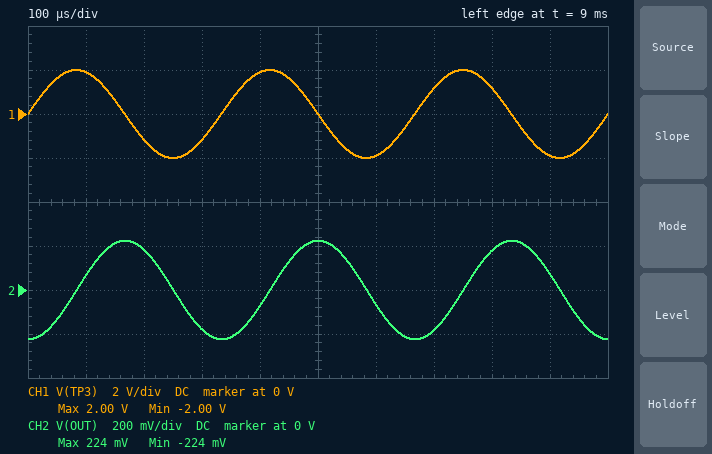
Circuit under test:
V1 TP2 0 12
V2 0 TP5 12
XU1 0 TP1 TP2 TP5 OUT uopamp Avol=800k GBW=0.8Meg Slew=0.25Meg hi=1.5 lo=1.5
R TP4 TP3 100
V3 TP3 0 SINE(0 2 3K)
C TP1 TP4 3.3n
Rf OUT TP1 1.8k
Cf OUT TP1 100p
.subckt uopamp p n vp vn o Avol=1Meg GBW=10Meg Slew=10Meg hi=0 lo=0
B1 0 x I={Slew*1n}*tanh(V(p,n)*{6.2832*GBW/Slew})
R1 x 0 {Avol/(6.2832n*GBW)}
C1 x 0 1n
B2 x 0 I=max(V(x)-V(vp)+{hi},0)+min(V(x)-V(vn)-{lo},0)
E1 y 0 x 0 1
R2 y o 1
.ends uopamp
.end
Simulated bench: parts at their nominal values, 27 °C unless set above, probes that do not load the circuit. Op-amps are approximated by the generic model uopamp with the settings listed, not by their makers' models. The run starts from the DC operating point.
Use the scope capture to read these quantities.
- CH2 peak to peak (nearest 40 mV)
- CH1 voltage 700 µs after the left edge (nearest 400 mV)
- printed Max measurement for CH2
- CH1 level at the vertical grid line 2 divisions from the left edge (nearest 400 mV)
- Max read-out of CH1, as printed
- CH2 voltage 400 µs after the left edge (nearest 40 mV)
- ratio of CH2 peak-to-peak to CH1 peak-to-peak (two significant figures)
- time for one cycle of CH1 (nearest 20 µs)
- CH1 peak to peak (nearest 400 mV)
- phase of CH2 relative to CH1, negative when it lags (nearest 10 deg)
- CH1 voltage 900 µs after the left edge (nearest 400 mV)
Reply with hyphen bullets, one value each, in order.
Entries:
- 440 mV
- 1.2 V
- 224 mV
- -1.2 V
- 2.00 V
- -80 mV
- 0.11
- 340 µs
- 4.0 V
- -90 deg
- -2.0 V
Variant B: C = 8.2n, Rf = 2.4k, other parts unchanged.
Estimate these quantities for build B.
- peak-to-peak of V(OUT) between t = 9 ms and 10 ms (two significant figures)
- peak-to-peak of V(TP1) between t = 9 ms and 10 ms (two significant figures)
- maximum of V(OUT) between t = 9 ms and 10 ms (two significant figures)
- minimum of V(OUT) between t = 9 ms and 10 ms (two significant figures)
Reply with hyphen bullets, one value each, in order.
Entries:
- 1.5 V
- 5.6 mV
- 740 mV
- -740 mV
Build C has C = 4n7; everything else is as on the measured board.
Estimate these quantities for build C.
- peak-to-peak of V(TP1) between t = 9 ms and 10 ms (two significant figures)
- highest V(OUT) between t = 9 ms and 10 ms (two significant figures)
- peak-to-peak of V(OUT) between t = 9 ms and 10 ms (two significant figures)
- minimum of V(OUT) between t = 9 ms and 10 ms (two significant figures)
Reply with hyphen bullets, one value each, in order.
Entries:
- 2.4 mV
- 320 mV
- 640 mV
- -320 mV
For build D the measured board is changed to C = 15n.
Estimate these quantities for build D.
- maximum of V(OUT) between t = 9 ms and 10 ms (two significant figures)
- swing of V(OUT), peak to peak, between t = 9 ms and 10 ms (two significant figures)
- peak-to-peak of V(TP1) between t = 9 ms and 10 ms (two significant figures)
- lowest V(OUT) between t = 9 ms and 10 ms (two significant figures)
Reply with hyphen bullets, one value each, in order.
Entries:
- 1.0 V
- 2.0 V
- 7.7 mV
- -1.0 V
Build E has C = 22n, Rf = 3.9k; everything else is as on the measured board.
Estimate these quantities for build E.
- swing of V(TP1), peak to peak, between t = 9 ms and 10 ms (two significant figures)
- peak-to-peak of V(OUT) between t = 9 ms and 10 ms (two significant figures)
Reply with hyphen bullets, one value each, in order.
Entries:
- 25 mV
- 6.5 V
